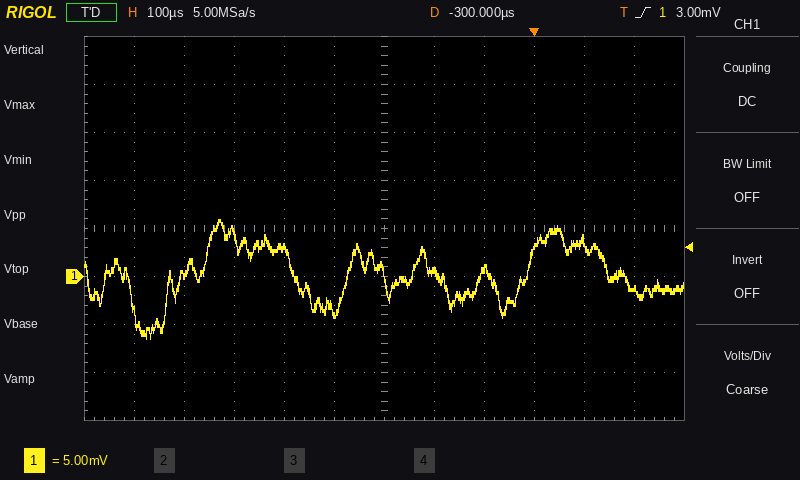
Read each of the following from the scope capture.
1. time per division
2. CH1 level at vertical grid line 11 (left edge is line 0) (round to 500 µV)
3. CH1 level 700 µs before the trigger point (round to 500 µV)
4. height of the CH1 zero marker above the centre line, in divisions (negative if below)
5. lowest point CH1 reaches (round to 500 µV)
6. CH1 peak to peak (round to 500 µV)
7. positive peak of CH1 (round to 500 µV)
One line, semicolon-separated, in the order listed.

100 µs; -1.5 mV; 0.0 mV; -1.0 div; -6.5 mV; 12.5 mV; 6.0 mV
